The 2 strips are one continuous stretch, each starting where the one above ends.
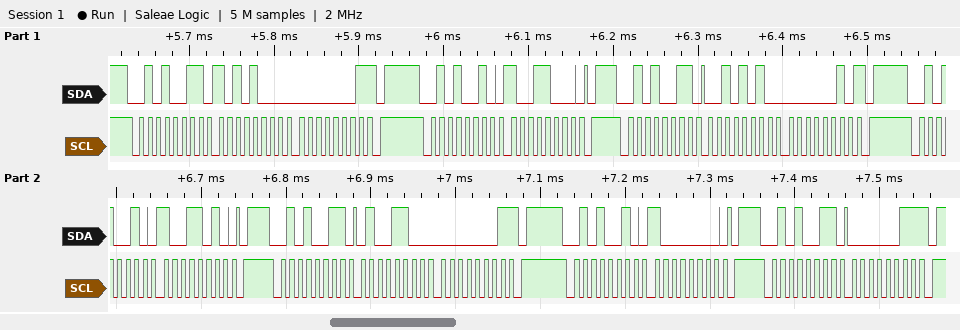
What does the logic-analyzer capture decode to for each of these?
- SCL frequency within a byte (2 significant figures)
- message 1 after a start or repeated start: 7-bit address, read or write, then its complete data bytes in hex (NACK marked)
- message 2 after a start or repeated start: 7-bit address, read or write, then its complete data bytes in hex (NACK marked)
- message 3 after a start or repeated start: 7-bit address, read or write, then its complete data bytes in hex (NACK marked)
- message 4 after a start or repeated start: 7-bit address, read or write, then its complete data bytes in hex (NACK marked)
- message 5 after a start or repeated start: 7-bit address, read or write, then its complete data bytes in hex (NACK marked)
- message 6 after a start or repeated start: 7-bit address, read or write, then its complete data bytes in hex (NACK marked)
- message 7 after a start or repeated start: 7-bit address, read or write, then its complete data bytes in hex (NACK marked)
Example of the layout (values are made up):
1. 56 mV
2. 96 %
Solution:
1. 100 kHz
2. 0x29 read: A8 01 NACK
3. 0x29 write: 98
4. 0x29 read: 2A 02 NACK
5. 0x29 write: 9A
6. 0x29 read: 4C 01 NACK
7. 0x29 write: 80
8. 0x29 read: 03 NACK
